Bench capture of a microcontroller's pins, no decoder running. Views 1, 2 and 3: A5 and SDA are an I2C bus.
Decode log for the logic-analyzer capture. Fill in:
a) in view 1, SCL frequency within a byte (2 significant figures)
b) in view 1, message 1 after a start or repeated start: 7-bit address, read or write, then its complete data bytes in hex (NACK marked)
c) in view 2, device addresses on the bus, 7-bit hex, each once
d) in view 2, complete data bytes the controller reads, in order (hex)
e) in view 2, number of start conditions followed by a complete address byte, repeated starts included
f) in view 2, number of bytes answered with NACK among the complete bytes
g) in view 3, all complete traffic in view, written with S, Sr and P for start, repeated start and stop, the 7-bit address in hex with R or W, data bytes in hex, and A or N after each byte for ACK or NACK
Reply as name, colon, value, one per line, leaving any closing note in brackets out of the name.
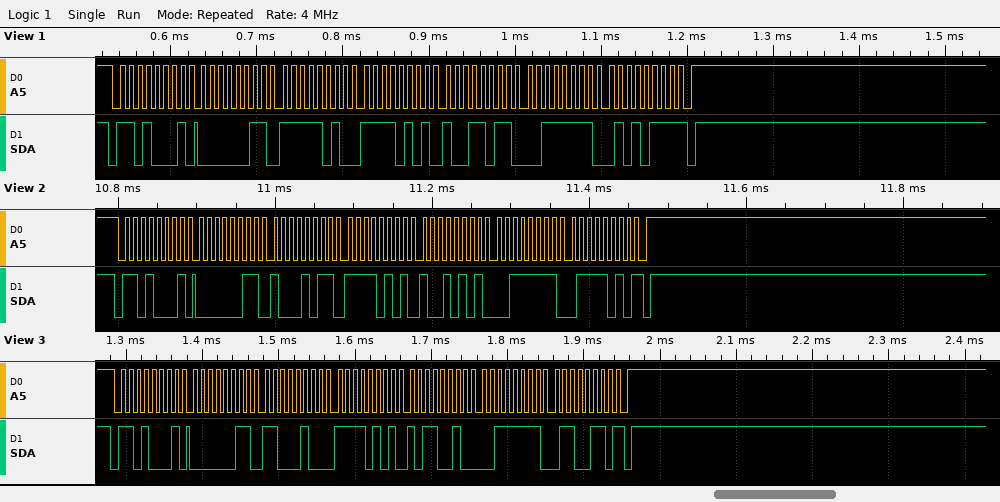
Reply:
in view 1, SCL frequency within a byte: 100 kHz
in view 1, message 1 after a start or repeated start: 7-bit address, read or write, then its complete data bytes in hex: 0x68 read: 03 FA F5 9B 3F 57 NACK
in view 2, device addresses on the bus, 7-bit hex, each once: 0x68
in view 2, complete data bytes the controller reads, in order: 03 8B F5 95 3F 7A
in view 2, number of start conditions followed by a complete address byte, repeated starts included: 1
in view 2, number of bytes answered with NACK among the complete bytes: 1
in view 3, all complete traffic in view, written with S, Sr and P for start, repeated start and stop, the 7-bit address in hex with R or W, data bytes in hex, and A or N after each byte for ACK or NACK: S 68R A 03 A C4 A F5 A B2 A 3F A 66 N P
